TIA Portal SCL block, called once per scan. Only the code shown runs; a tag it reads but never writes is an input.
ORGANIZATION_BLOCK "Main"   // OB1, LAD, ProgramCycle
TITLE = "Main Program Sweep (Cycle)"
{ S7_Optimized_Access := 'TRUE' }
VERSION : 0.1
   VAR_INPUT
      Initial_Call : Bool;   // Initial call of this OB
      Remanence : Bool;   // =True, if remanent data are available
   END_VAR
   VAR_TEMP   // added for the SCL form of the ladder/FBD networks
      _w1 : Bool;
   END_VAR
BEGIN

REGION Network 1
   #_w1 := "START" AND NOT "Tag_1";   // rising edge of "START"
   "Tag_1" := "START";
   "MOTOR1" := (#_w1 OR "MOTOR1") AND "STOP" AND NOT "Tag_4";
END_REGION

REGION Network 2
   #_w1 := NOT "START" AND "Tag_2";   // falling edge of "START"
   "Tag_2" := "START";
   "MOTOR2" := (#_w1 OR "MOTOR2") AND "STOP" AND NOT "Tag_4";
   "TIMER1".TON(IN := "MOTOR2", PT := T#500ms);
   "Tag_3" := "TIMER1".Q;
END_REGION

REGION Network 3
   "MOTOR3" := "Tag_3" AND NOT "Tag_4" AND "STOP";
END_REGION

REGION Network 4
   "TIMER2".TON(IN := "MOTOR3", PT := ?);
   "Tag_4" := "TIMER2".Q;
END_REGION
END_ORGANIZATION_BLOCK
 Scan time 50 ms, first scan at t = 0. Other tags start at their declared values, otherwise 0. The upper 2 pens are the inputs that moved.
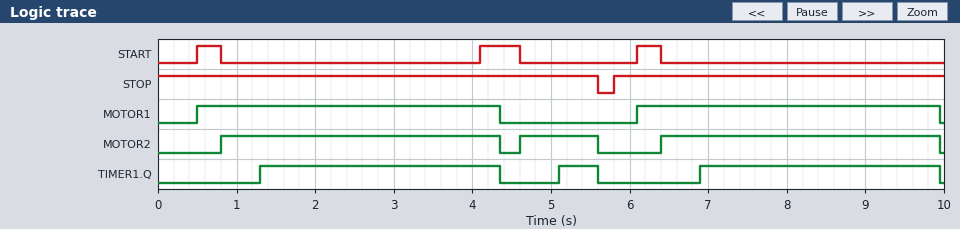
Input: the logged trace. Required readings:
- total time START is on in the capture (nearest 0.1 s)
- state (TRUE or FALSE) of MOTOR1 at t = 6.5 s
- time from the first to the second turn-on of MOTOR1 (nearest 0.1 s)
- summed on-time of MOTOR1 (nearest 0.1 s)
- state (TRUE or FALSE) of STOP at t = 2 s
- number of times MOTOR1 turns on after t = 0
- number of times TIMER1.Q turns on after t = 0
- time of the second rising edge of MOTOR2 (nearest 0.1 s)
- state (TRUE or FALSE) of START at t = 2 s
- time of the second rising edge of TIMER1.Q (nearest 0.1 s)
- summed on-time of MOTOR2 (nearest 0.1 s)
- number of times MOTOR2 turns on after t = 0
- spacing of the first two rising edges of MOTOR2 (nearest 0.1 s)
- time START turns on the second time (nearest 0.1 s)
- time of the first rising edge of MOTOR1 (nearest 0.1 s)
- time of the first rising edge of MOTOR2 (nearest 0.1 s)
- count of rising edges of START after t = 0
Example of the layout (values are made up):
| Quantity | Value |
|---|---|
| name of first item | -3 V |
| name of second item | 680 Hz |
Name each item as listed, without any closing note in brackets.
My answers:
| Quantity | Value |
|---|---|
| total time START is on in the capture | 1.1 s |
| state (TRUE or FALSE) of MOTOR1 at t = 6.5 s | TRUE |
| time from the first to the second turn-on of MOTOR1 | 5.6 s |
| summed on-time of MOTOR1 | 7.7 s |
| state (TRUE or FALSE) of STOP at t = 2 s | TRUE |
| number of times MOTOR1 turns on after t = 0 | 2 |
| number of times TIMER1.Q turns on after t = 0 | 3 |
| time of the second rising edge of MOTOR2 | 4.6 s |
| state (TRUE or FALSE) of START at t = 2 s | FALSE |
| time of the second rising edge of TIMER1.Q | 5.1 s |
| summed on-time of MOTOR2 | 8.1 s |
| number of times MOTOR2 turns on after t = 0 | 3 |
| spacing of the first two rising edges of MOTOR2 | 3.8 s |
| time START turns on the second time | 4.1 s |
| time of the first rising edge of MOTOR1 | 0.5 s |
| time of the first rising edge of MOTOR2 | 0.8 s |
| count of rising edges of START after t = 0 | 3 |
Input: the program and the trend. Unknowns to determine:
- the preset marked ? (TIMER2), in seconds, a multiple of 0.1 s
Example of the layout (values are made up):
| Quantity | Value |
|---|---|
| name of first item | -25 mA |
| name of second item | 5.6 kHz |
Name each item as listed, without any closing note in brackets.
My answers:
| Quantity | Value |
|---|---|
| the preset marked ? (TIMER2), in seconds, a multiple of 0.1 s | 3.0 s |
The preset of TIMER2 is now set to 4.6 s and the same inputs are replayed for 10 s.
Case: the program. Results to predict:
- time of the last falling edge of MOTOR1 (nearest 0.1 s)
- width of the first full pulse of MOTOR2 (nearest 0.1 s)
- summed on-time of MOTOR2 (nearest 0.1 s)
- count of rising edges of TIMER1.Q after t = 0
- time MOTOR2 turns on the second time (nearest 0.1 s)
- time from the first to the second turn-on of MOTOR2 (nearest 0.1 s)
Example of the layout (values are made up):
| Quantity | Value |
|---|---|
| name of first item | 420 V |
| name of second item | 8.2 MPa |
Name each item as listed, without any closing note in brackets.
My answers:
| Quantity | Value |
|---|---|
| time of the last falling edge of MOTOR1 | 5.6 s |
| width of the first full pulse of MOTOR2 | 4.8 s |
| summed on-time of MOTOR2 | 8.4 s |
| count of rising edges of TIMER1.Q after t = 0 | 2 |
| time MOTOR2 turns on the second time | 6.4 s |
| time from the first to the second turn-on of MOTOR2 | 5.6 s |
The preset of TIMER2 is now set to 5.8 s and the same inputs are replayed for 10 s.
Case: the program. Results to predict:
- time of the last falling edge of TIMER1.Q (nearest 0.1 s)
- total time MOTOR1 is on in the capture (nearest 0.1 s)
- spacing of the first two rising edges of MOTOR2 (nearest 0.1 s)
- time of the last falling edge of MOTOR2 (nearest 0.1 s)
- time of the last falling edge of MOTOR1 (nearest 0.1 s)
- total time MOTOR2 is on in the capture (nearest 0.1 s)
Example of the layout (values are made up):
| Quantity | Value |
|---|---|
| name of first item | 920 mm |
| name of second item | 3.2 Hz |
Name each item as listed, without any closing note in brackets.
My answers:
| Quantity | Value |
|---|---|
| time of the last falling edge of TIMER1.Q | 5.6 s |
| total time MOTOR1 is on in the capture | 9.0 s |
| spacing of the first two rising edges of MOTOR2 | 5.6 s |
| time of the last falling edge of MOTOR2 | 5.6 s |
| time of the last falling edge of MOTOR1 | 5.6 s |
| total time MOTOR2 is on in the capture | 8.4 s |
